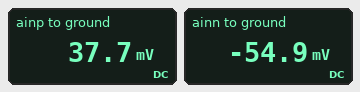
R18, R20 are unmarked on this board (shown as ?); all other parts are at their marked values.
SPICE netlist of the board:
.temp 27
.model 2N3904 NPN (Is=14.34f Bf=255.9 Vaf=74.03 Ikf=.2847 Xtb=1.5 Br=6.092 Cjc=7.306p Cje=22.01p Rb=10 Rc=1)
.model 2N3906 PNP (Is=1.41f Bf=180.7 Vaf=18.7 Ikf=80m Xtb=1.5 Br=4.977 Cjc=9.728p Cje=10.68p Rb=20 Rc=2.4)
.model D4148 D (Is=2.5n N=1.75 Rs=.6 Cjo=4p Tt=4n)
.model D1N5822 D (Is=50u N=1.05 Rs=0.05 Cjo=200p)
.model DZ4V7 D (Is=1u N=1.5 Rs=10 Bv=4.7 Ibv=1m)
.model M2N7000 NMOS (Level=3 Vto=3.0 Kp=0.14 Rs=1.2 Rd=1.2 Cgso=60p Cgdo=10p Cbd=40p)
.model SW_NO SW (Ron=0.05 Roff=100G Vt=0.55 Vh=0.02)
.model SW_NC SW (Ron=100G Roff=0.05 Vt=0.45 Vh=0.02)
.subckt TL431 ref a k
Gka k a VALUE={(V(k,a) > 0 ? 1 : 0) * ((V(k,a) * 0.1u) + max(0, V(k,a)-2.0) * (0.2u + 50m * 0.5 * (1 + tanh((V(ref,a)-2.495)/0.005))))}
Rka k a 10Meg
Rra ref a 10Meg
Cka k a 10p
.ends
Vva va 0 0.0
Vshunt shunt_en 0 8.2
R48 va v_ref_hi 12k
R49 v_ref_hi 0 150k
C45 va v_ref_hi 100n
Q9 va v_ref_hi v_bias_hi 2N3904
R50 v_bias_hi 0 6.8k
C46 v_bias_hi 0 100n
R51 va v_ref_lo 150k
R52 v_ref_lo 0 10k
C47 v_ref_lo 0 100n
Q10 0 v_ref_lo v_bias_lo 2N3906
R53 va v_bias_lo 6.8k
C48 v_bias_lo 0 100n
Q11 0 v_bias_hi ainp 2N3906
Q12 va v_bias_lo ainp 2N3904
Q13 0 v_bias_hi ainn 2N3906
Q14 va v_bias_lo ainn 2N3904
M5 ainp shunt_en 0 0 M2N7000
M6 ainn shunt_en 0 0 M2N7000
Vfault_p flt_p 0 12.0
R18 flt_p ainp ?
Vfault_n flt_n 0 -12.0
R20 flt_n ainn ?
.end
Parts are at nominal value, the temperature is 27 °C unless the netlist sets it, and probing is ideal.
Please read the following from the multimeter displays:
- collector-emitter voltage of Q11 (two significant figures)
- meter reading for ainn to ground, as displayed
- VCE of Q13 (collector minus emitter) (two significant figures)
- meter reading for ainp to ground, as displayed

-38 mV
-54.9 mV
55 mV
37.7 mV
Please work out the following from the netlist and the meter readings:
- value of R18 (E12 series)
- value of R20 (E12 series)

1.2 kΩ
820 Ω
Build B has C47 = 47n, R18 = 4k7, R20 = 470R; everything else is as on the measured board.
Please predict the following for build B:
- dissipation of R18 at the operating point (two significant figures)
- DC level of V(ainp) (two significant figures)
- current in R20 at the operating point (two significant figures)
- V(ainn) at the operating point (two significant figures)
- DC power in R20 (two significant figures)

31 mW
9.6 mV
25 mA
-95 mV
300 mW
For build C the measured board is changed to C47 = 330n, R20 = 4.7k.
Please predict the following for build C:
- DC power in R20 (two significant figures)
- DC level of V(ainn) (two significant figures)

31 mW
-9.6 mV
